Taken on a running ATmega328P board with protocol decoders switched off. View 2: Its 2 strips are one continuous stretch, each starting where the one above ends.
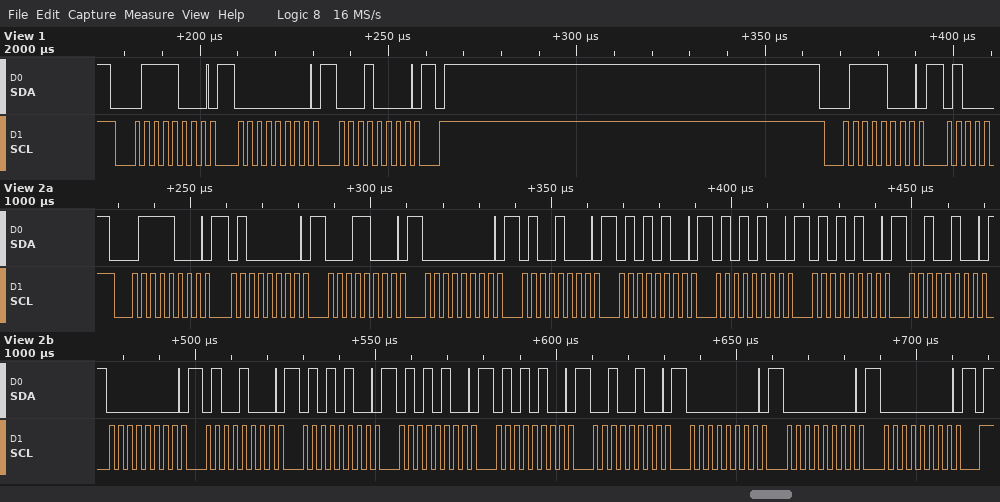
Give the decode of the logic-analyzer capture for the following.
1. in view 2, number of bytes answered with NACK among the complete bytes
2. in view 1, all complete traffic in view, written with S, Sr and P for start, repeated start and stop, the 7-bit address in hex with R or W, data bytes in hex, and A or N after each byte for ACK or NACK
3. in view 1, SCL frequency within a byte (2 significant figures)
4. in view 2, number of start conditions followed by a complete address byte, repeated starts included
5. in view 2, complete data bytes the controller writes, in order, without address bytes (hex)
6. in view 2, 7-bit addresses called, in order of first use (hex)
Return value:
0
S 3CW A 00 A 10 A P S 3CW A
400 kHz
1
40 18 00 48 54 54 54 24 00 48 54 54 54 24 00 00 00
0x3C
